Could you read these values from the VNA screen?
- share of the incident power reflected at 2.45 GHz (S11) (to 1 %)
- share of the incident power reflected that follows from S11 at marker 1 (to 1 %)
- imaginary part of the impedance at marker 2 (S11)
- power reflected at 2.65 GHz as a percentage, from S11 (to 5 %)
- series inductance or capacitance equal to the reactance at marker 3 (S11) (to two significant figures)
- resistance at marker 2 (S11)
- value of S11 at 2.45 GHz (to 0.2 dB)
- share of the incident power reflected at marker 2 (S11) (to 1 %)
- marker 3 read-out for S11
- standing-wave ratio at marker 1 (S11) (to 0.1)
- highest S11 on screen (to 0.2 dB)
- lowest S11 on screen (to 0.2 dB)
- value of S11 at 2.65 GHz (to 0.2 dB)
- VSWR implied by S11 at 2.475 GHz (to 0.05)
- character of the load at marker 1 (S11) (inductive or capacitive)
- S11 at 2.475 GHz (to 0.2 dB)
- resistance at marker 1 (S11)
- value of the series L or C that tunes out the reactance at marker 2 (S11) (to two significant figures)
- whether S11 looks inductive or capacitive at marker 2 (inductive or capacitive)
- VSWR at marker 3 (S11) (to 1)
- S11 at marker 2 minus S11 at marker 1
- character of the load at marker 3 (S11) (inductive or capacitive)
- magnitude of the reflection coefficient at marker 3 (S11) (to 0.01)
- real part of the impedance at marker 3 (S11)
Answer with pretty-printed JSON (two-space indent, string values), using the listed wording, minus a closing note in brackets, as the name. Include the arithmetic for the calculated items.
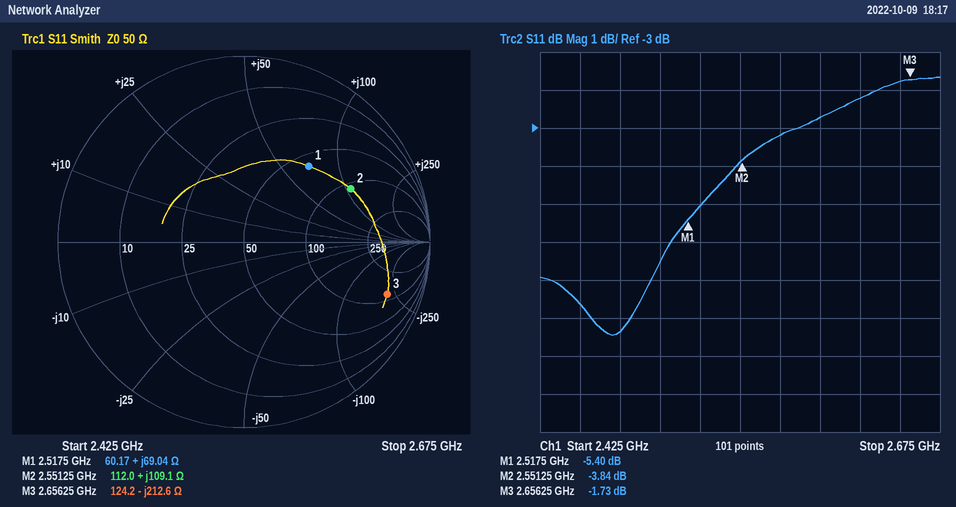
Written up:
{
  "share of the incident power reflected at 2.45 GHz (S11)": "10^(-7.6/10) ≈ 17 %",
  "share of the incident power reflected that follows from S11 at marker 1": "10^(-5.4/10) ≈ 29 %",
  "imaginary part of the impedance at marker 2": "+109.1 Ω",
  "power reflected at 2.65 GHz as a percentage, from S11": "10^(-1.8/10) ≈ 66.1 %, so 65 % to the nearest 5 %",
  "series inductance or capacitance equal to the reactance at marker 3 (S11)": "C = 1/(2π × 2.65625 GHz × 212.6 Ω) ≈ 282 fF, so 280 fF to two significant figures",
  "resistance at marker 2": "112.0 Ω",
  "value of S11 at 2.45 GHz": "-7.6 dB",
  "share of the incident power reflected at marker 2 (S11)": "10^(-3.84/10) ≈ 41 %",
  "marker 3 read-out for S11": "-1.73 dB",
  "standing-wave ratio at marker 1 (S11)": "3.3",
  "highest S11 on screen": "-1.6 dB",
  "lowest S11 on screen": "-8.4 dB",
  "value of S11 at 2.65 GHz": "-1.8 dB",
  "VSWR implied by S11 at 2.475 GHz": "|Γ| = 10^(-8.4/20) = 0.3802; VSWR = (1 + 0.3802)/(1 − 0.3802) ≈ 2.23, so 2.25 to the nearest 0.05",
  "character of the load at marker 1 (S11)": "inductive",
  "S11 at 2.475 GHz": "-8.4 dB",
  "resistance at marker 1": "60.17 Ω",
  "value of the series L or C that tunes out the reactance at marker 2 (S11)": "C = 1/(2π × 2.55125 GHz × 109.1 Ω) ≈ 572 fF, so 570 fF to two significant figures",
  "whether S11 looks inductive or capacitive at marker 2": "inductive",
  "VSWR at marker 3 (S11)": "10",
  "S11 at marker 2 minus S11 at marker 1": "-3.84 − (-5.4) = 1.56 dB",
  "character of the load at marker 3 (S11)": "capacitive",
  "magnitude of the reflection coefficient at marker 3 (S11)": "10^(-1.73/20) ≈ 0.82",
  "real part of the impedance at marker 3": "124.2 Ω"
}
